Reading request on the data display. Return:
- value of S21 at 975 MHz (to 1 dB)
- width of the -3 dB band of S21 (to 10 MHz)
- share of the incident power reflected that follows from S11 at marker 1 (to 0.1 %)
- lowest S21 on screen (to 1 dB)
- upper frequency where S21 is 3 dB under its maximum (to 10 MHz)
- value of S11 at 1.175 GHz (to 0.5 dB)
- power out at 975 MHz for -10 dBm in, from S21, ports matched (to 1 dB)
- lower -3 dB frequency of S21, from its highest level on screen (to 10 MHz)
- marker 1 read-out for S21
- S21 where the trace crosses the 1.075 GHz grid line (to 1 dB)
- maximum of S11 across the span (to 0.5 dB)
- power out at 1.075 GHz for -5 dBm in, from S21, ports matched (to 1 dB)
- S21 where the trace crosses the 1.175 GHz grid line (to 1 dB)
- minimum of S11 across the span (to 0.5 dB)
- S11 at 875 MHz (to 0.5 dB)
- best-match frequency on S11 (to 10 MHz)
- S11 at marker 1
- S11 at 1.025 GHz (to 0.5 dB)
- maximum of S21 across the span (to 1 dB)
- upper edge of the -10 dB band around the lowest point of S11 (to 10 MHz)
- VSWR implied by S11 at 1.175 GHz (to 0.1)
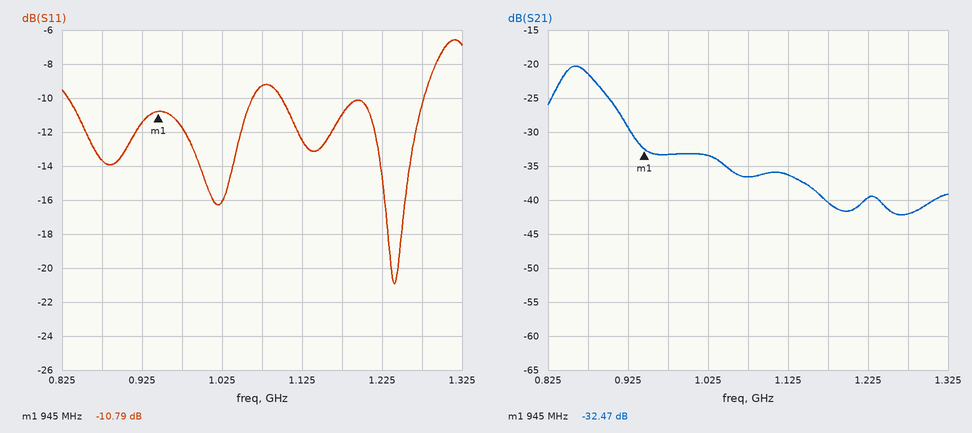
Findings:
-33 dB
50 MHz
8.3 %
-42 dB
890 MHz
-11.0 dB
-43 dBm
840 MHz
-32.47 dB
-37 dB
-6.5 dB
-42 dBm
-40 dB
-21.0 dB
-13.5 dB
1.24 GHz
-10.79 dB
-16.0 dB
-20 dB
1.28 GHz
1.8
